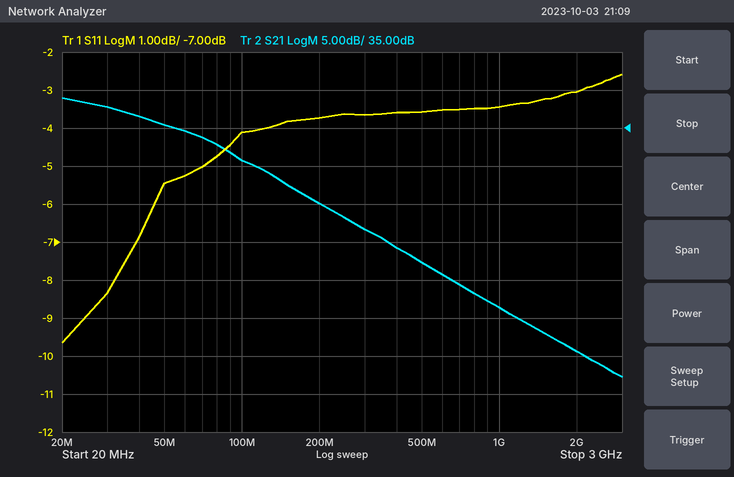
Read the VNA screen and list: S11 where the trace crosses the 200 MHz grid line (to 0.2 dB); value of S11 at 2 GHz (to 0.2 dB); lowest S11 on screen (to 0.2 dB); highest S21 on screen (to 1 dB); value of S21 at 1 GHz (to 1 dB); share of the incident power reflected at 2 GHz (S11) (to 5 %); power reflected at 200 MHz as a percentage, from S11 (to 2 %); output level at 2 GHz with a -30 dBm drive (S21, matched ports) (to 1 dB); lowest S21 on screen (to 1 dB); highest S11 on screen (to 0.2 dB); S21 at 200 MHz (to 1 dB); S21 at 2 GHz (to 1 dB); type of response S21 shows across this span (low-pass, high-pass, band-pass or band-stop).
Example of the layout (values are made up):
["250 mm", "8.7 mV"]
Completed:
["-3.8 dB", "-3.0 dB", "-9.6 dB", "39 dB", "11 dB", "50 %", "42 %", "-24 dBm", "2 dB", "-2.6 dB", "25 dB", "6 dB", "low-pass"]
